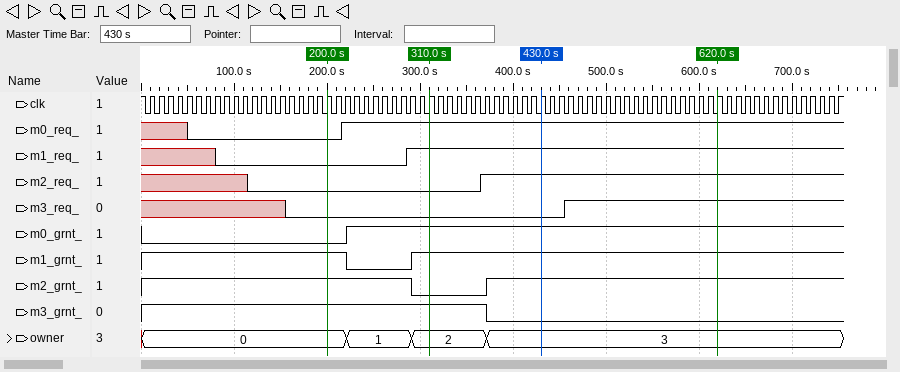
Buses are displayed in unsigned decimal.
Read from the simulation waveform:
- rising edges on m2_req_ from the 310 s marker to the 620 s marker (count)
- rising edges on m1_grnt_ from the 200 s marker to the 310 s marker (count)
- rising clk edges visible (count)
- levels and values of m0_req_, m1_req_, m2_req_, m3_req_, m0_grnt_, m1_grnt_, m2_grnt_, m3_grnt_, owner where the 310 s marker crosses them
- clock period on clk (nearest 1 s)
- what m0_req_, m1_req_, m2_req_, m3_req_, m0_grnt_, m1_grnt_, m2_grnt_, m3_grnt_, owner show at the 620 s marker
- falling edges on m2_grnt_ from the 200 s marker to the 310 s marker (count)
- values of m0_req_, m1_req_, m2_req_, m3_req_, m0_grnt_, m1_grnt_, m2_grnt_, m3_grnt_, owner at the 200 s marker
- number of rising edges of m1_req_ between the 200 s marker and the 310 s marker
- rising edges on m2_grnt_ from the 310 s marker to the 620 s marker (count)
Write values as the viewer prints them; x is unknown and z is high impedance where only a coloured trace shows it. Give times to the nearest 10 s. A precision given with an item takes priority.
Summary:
1
1
75
m0_req_=1, m1_req_=1, m2_req_=0, m3_req_=0, m0_grnt_=1, m1_grnt_=1, m2_grnt_=0, m3_grnt_=1, owner=2
10 s
m0_req_=1, m1_req_=1, m2_req_=1, m3_req_=1, m0_grnt_=1, m1_grnt_=1, m2_grnt_=1, m3_grnt_=0, owner=3
1
m0_req_=0, m1_req_=0, m2_req_=0, m3_req_=0, m0_grnt_=0, m1_grnt_=1, m2_grnt_=1, m3_grnt_=1, owner=0
1
1
